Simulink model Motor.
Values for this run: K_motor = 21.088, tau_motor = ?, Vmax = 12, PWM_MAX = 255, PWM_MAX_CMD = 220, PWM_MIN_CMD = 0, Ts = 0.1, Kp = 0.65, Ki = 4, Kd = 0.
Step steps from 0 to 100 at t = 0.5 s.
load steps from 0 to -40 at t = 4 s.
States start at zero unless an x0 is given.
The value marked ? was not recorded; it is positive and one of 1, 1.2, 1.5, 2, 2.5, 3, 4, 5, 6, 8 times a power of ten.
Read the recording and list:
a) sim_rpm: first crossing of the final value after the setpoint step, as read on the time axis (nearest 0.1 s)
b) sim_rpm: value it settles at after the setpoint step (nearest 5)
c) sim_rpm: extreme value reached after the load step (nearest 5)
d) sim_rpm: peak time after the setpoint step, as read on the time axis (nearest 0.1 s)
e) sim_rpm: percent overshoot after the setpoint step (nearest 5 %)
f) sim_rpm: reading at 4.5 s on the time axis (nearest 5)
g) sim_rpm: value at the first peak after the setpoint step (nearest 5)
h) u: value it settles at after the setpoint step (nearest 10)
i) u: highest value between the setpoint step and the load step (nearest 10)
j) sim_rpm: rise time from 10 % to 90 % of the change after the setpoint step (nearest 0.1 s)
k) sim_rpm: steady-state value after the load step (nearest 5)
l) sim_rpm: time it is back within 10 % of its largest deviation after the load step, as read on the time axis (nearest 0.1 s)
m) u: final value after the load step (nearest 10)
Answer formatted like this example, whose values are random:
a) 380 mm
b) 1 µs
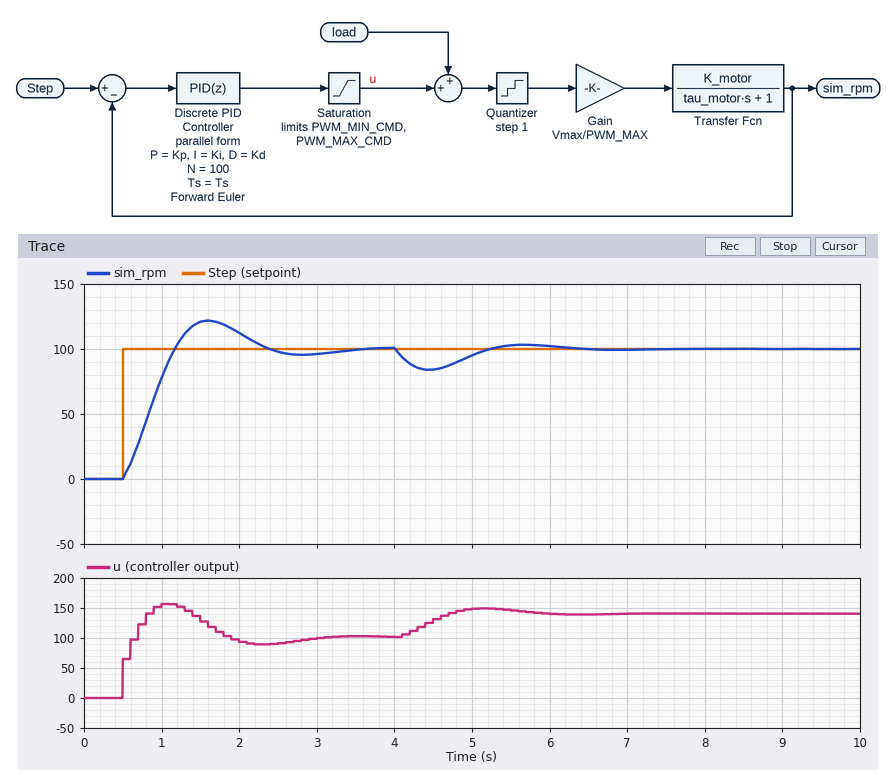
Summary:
a) 1.2 s
b) 100
c) 85
d) 1.6 s
e) 20 %
f) 85
g) 120
h) 100
i) 160
j) 0.5 s
k) 100
l) 6.1 s
m) 140
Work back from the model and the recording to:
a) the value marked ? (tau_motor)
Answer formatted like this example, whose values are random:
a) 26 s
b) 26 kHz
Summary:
a) 0.5
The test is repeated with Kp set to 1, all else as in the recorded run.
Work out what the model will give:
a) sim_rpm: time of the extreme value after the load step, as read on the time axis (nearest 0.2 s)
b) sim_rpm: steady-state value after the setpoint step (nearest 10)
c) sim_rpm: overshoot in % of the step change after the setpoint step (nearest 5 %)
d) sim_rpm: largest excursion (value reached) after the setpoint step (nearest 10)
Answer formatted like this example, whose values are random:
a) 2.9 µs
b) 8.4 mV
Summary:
a) 4.4 s
b) 100
c) 15 %
d) 110
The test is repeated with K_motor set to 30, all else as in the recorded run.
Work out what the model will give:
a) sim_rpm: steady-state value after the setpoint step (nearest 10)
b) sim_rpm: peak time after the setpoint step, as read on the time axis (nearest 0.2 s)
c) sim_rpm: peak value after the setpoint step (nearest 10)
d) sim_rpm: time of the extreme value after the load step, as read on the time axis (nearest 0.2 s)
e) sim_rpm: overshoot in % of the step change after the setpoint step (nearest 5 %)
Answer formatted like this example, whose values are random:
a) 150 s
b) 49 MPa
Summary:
a) 100
b) 1.4 s
c) 130
d) 4.4 s
e) 25 %
